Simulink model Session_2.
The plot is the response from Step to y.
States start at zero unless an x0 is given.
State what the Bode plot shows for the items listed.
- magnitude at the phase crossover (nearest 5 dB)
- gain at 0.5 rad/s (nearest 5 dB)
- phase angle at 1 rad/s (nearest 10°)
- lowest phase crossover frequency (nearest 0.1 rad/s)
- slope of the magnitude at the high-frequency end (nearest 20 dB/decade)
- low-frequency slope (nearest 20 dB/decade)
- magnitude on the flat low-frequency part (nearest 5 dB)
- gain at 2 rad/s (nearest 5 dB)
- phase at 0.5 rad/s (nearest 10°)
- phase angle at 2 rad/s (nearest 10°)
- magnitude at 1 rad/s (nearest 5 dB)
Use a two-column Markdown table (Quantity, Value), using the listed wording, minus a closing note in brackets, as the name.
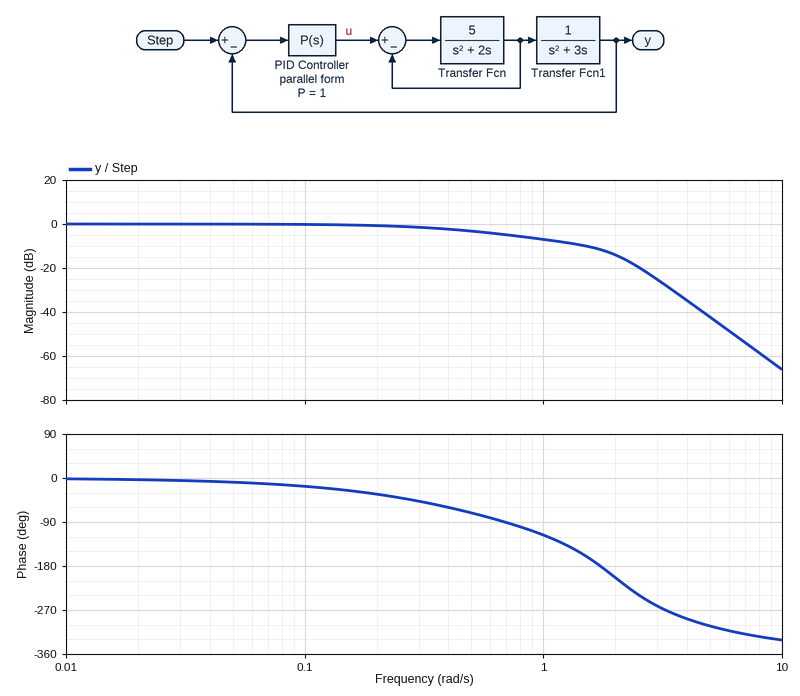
| Quantity | Value |
|---|---|
| magnitude at the phase crossover | -10 dB |
| gain at 0.5 rad/s | -5 dB |
| phase angle at 1 rad/s | -120° |
| lowest phase crossover frequency | 1.7 rad/s |
| slope of the magnitude at the high-frequency end | -80 dB/decade |
| low-frequency slope | 0 dB/decade |
| magnitude on the flat low-frequency part | 0 dB |
| gain at 2 rad/s | -15 dB |
| phase at 0.5 rad/s | -70° |
| phase angle at 2 rad/s | -200° |
| magnitude at 1 rad/s | -5 dB |
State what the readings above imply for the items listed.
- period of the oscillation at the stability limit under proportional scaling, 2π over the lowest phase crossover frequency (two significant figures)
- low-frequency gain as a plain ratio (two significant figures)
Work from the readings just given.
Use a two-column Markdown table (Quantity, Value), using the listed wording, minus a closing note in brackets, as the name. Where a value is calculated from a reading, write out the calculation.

| Quantity | Value |
|---|---|
| period of the oscillation at the stability limit under proportional scaling, 2π over the lowest phase crossover frequency | 2π / 1.7 = 3.7 s |
| low-frequency gain as a plain ratio | 10^(0 / 20) = 1.0 |
